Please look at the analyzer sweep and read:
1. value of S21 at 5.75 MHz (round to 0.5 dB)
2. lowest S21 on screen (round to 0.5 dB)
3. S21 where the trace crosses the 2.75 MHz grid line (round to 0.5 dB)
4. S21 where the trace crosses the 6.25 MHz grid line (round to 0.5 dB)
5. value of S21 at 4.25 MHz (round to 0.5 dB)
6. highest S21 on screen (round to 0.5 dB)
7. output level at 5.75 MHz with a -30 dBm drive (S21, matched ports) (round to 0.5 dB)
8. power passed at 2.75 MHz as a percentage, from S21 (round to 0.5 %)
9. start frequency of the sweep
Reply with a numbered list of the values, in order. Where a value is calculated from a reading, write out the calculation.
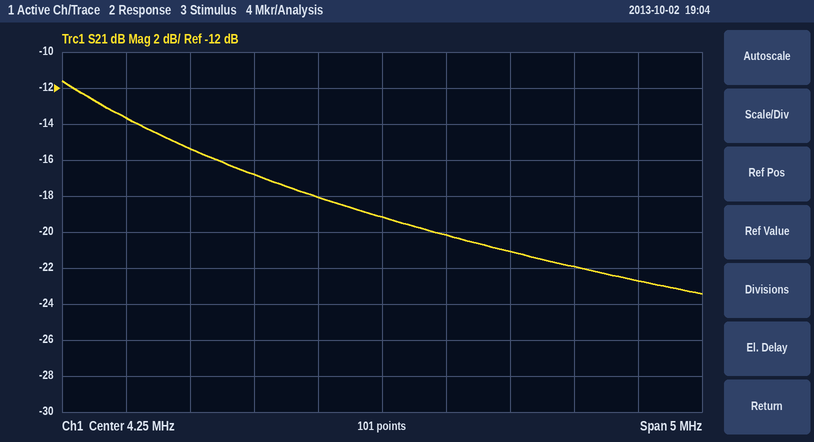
1. -22.0 dB
2. -23.5 dB
3. -15.5 dB
4. -22.5 dB
5. -19.0 dB
6. -11.5 dB
7. -30 dBm + (-22.0 dB) = -52.0 dBm
8. 10^(-15.5/10) ≈ 2.82 %, so 3.0 % to the nearest 0.5 %
9. 1.75 MHz
